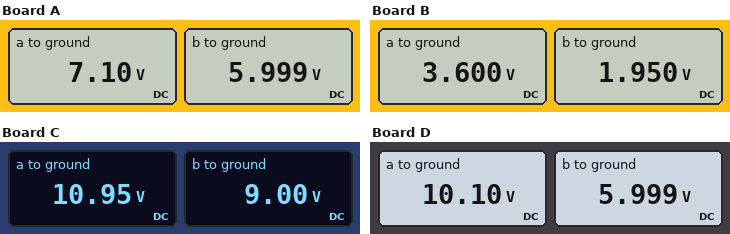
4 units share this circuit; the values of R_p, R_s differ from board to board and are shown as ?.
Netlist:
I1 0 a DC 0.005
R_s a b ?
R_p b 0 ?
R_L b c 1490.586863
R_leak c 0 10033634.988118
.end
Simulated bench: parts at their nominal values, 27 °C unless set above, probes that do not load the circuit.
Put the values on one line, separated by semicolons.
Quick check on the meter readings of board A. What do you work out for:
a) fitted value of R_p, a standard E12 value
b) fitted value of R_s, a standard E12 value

1.2 kΩ; 220 Ω
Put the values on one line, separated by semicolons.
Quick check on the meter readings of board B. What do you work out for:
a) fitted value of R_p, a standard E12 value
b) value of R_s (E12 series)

390 Ω; 330 Ω
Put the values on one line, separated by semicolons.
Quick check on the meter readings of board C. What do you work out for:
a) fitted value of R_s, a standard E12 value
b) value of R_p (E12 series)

390 Ω; 1.8 kΩ
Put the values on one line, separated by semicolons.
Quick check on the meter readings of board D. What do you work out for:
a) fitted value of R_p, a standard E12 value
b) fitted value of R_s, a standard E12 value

1.2 kΩ; 820 Ω
